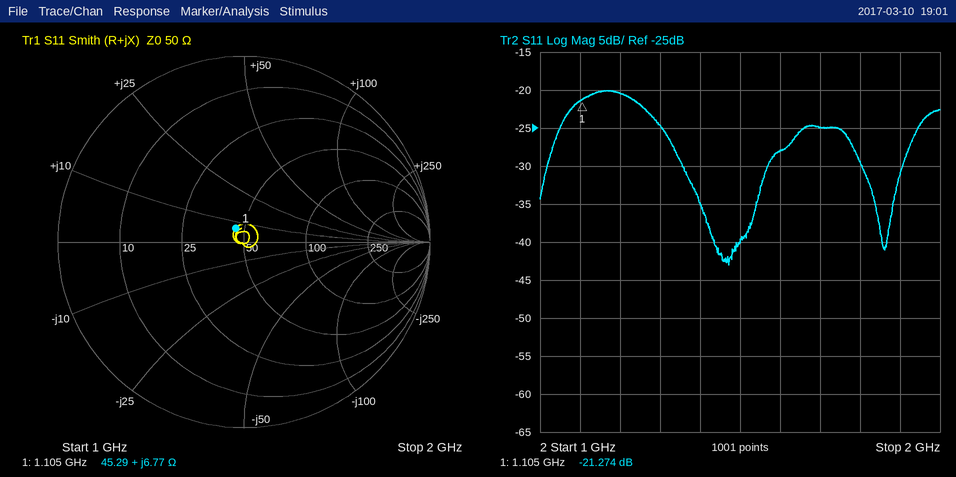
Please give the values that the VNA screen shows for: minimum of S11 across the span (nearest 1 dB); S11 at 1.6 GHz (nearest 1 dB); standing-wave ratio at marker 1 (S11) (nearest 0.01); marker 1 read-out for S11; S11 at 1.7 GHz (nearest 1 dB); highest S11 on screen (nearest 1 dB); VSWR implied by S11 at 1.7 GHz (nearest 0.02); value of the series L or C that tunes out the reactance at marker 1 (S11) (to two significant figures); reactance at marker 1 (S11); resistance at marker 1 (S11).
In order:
-43 dB
-28 dB
1.19
-21.274 dB
-25 dB
-20 dB
1.12
21 pF
+6.77 Ω
45.29 Ω
